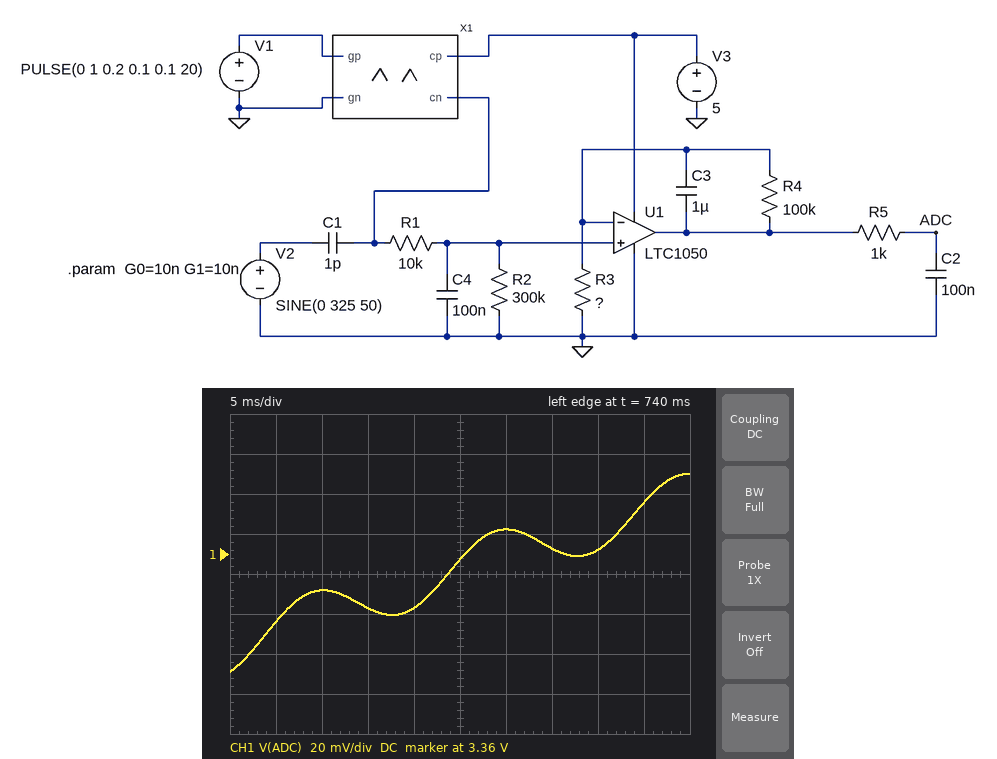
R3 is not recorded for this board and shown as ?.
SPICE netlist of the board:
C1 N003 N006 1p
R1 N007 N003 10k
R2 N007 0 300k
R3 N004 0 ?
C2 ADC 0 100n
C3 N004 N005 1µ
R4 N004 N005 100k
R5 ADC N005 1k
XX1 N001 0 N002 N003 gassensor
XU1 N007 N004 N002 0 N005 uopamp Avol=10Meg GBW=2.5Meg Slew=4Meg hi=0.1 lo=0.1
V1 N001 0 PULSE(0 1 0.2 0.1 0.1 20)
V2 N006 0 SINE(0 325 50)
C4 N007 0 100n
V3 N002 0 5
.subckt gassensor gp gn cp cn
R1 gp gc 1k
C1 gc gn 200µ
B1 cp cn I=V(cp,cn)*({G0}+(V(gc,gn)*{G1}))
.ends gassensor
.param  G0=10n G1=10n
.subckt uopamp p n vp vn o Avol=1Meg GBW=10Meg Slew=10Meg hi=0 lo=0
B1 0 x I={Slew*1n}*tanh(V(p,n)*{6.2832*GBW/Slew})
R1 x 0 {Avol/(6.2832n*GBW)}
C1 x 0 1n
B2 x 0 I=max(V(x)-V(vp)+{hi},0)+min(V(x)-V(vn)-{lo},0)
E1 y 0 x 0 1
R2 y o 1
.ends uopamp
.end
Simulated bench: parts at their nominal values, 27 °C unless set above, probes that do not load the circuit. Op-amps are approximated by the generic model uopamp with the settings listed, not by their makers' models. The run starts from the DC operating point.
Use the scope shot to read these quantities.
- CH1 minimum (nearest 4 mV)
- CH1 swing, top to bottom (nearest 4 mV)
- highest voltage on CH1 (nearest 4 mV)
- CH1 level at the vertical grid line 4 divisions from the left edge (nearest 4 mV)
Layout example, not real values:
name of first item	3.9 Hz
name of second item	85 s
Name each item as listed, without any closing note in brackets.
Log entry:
CH1 minimum	3.300 V
CH1 swing, top to bottom	100 mV
highest voltage on CH1	3.400 V
CH1 level at the vertical grid line 4 divisions from the left edge	3.332 V
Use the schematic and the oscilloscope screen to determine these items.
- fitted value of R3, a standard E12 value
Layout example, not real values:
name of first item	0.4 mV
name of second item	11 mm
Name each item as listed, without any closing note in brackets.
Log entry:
fitted value of R3, a standard E12 value	820 Ω
